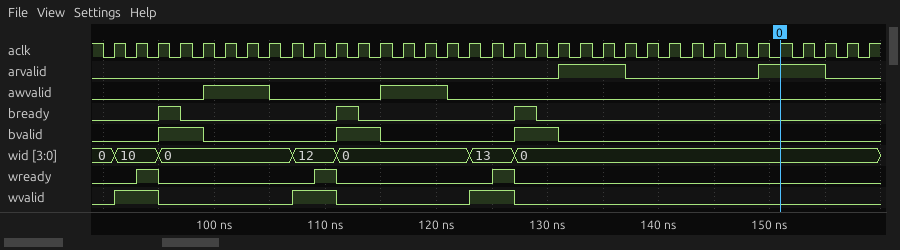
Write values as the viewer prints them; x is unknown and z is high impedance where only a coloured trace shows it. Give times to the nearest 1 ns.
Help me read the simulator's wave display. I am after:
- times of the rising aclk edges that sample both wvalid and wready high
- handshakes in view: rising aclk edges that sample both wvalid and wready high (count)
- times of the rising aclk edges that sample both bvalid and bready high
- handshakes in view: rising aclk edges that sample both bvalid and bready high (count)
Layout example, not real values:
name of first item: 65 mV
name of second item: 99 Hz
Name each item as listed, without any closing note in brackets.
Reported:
times of the rising aclk edges that sample both wvalid and wready high: 95 ns, 111 ns, 127 ns
handshakes in view: rising aclk edges that sample both wvalid and wready high: 3
times of the rising aclk edges that sample both bvalid and bready high: 97 ns, 113 ns, 129 ns
handshakes in view: rising aclk edges that sample both bvalid and bready high: 3
